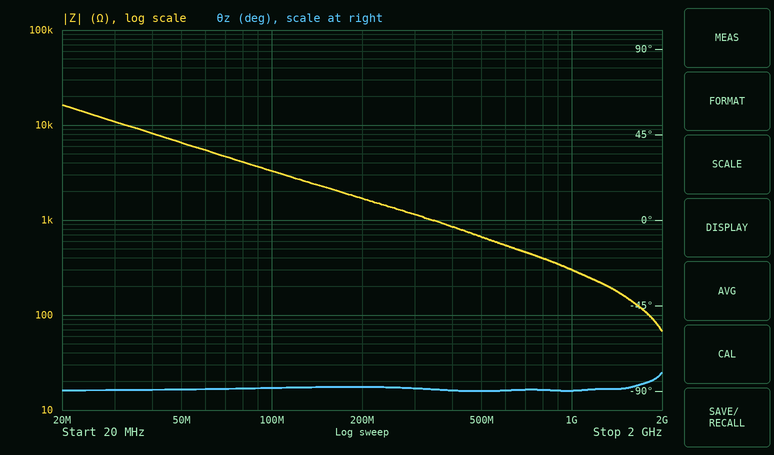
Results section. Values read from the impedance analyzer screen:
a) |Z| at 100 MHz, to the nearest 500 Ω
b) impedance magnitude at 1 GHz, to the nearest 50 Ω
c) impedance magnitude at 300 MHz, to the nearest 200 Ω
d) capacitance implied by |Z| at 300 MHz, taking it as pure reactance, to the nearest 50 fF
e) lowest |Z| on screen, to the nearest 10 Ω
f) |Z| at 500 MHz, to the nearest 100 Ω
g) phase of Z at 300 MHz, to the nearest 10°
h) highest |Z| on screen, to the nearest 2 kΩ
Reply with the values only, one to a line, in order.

3.5 kΩ
300 Ω
1.2 kΩ
450 fF
70 Ω
700 Ω
-90°
16 kΩ
